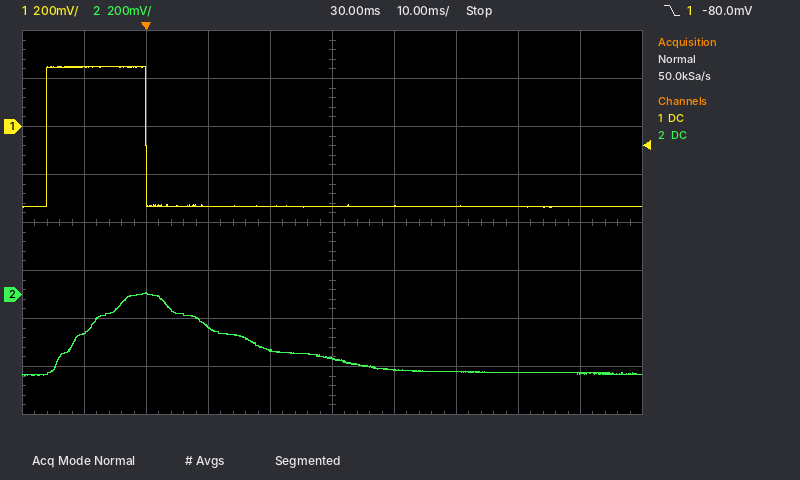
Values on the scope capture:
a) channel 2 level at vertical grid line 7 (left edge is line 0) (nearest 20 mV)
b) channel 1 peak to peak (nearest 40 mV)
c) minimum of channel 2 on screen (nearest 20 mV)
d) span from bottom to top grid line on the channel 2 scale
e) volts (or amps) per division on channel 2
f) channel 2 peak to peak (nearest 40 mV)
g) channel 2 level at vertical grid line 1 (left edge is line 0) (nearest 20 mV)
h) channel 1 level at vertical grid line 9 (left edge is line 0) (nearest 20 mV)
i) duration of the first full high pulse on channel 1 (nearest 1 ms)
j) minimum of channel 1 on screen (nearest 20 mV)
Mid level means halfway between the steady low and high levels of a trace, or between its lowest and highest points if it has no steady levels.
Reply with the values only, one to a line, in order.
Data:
-320 mV
600 mV
-340 mV
1.6 V
200 mV
360 mV
-160 mV
-340 mV
16 ms
-340 mV
